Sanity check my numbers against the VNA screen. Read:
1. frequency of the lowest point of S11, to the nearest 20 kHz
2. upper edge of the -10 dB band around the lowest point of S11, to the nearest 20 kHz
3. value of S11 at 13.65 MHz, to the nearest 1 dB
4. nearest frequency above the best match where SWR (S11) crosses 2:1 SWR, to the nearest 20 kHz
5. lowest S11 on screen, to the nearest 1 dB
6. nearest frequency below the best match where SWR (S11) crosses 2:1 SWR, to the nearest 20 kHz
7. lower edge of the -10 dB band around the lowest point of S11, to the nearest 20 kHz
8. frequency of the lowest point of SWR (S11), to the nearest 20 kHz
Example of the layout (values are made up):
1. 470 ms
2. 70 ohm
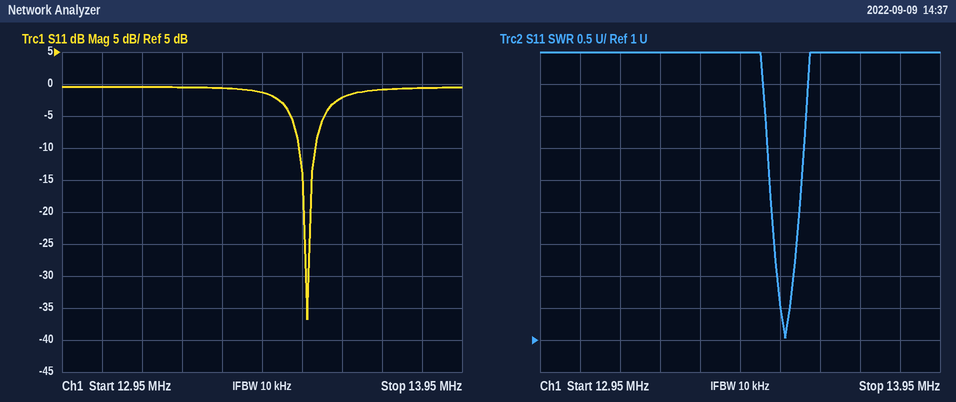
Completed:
1. 13.56 MHz
2. 13.58 MHz
3. -2 dB
4. 13.58 MHz
5. -37 dB
6. 13.54 MHz
7. 13.54 MHz
8. 13.56 MHz
